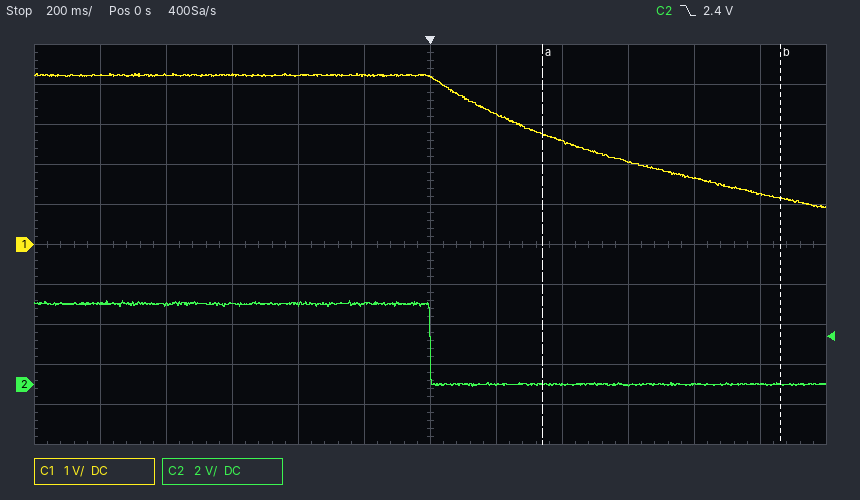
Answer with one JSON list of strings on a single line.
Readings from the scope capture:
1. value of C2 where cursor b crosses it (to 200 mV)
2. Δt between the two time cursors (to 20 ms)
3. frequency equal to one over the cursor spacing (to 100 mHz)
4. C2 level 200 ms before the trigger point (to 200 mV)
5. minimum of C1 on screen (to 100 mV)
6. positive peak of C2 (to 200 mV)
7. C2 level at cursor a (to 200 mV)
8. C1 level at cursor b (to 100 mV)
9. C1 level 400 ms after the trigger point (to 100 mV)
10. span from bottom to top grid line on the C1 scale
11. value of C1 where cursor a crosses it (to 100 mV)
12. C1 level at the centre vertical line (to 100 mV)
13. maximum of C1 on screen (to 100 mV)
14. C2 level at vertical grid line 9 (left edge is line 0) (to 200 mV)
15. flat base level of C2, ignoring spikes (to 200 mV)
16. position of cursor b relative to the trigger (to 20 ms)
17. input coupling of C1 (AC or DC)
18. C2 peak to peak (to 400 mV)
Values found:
["0.0 V", "720 ms", "1.4 Hz", "4.0 V", "900 mV", "4.2 V", "0.0 V", "1.2 V", "2.6 V", "10 V", "2.8 V", "4.2 V", "4.3 V", "0.0 V", "0.0 V", "+1.06 s", "DC", "4.4 V"]
